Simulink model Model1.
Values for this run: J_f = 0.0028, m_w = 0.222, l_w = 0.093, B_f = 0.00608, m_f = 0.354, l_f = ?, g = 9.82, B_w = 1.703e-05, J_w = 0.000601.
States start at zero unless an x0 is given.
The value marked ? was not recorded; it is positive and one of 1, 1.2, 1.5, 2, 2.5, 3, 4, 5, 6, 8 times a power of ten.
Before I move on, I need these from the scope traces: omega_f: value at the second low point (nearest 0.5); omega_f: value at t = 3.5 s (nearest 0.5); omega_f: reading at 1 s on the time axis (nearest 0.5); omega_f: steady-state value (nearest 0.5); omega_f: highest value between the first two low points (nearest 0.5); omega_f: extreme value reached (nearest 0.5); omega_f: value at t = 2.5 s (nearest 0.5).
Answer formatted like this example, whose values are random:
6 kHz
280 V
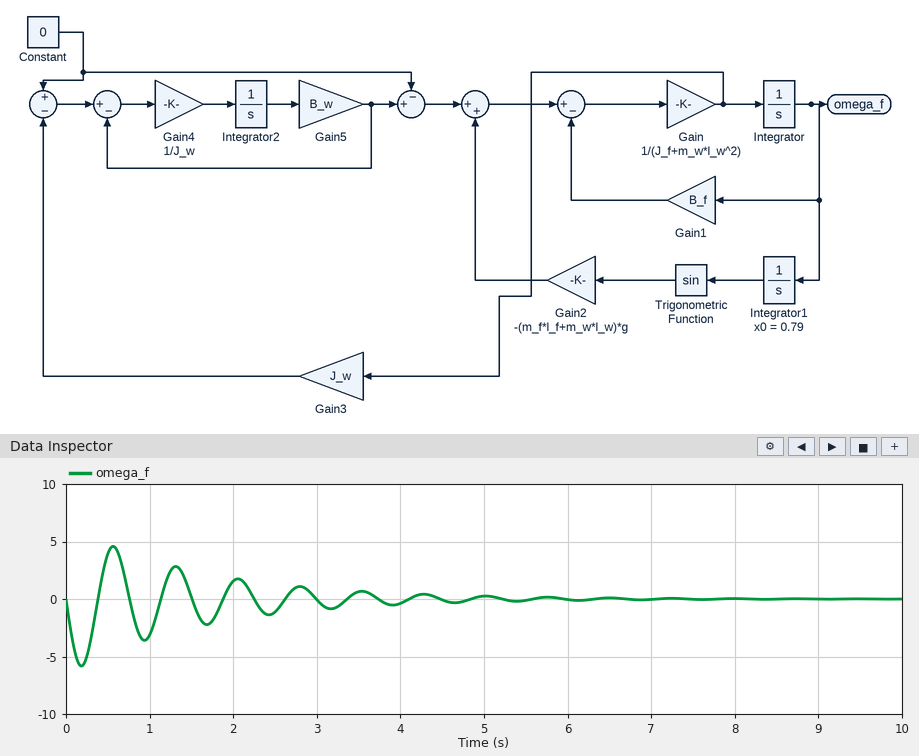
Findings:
-3.5
0.5
-3.0
0.0
4.5
-6.0
-1.0
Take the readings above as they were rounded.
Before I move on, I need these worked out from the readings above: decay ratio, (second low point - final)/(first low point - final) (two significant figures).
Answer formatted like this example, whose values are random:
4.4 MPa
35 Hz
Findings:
0.58
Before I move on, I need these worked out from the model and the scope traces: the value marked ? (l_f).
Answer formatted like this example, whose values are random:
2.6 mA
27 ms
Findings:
0.04
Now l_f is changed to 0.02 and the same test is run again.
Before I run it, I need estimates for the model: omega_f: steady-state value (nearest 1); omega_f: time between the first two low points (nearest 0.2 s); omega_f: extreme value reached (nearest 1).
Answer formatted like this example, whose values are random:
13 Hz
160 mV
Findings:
0
0.8 s
-5
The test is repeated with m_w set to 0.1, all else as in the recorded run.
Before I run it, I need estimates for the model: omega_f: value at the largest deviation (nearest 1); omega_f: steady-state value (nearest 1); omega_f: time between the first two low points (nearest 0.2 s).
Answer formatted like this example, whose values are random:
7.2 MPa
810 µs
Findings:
-5
0
0.8 s
